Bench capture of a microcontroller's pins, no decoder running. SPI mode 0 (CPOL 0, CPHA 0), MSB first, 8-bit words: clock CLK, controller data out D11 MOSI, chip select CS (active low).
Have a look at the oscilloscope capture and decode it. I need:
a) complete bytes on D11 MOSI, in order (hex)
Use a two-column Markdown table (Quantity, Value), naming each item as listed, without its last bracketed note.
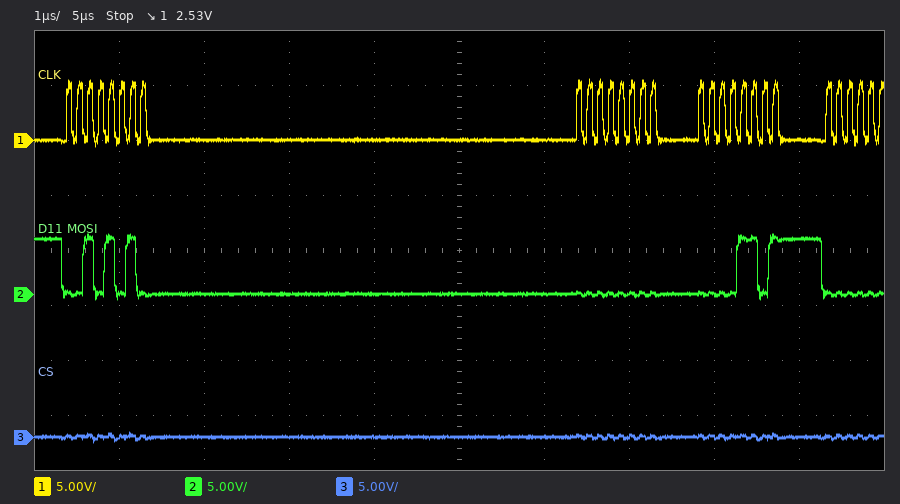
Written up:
| Quantity | Value |
|---|---|
| complete bytes on D11 MOSI, in order | 2A 00 0D |
